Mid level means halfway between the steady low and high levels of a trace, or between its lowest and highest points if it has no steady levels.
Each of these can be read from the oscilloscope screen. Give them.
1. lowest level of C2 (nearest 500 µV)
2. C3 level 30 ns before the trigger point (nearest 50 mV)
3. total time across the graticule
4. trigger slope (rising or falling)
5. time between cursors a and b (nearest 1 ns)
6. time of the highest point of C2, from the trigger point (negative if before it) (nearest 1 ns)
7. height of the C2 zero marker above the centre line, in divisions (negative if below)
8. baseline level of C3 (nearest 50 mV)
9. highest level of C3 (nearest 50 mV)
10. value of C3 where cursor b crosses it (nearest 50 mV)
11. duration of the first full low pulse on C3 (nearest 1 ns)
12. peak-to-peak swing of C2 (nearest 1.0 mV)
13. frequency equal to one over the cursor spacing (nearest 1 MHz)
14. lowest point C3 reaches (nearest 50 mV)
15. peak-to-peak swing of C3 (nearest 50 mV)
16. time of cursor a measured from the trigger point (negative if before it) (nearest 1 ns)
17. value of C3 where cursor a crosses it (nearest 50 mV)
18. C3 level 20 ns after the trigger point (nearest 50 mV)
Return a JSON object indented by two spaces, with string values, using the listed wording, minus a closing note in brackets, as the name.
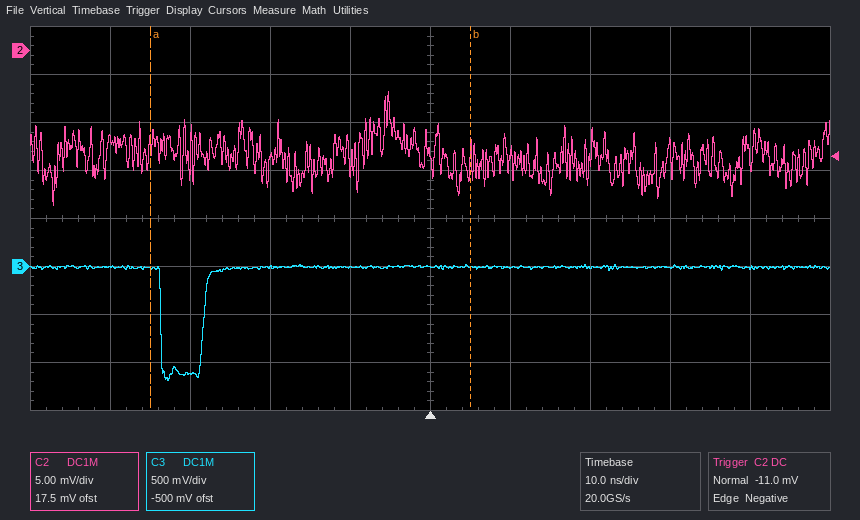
{
  "lowest level of C2": "-16.0 mV",
  "C3 level 30 ns before the trigger point": "-1.10 V",
  "total time across the graticule": "100 ns",
  "trigger slope": "falling",
  "time between cursors a and b": "40 ns",
  "time of the highest point of C2, from the trigger point (negative if before it)": "-5 ns",
  "height of the C2 zero marker above the centre line, in divisions": "+3.5 div",
  "baseline level of C3": "0 mV",
  "highest level of C3": "0 mV",
  "value of C3 where cursor b crosses it": "0 mV",
  "duration of the first full low pulse on C3": "5 ns",
  "peak-to-peak swing of C2": "12.0 mV",
  "frequency equal to one over the cursor spacing": "25 MHz",
  "lowest point C3 reaches": "-1.20 V",
  "peak-to-peak swing of C3": "1.20 V",
  "time of cursor a measured from the trigger point (negative if before it)": "-35 ns",
  "value of C3 where cursor a crosses it": "0 mV",
  "C3 level 20 ns after the trigger point": "0 mV"
}
